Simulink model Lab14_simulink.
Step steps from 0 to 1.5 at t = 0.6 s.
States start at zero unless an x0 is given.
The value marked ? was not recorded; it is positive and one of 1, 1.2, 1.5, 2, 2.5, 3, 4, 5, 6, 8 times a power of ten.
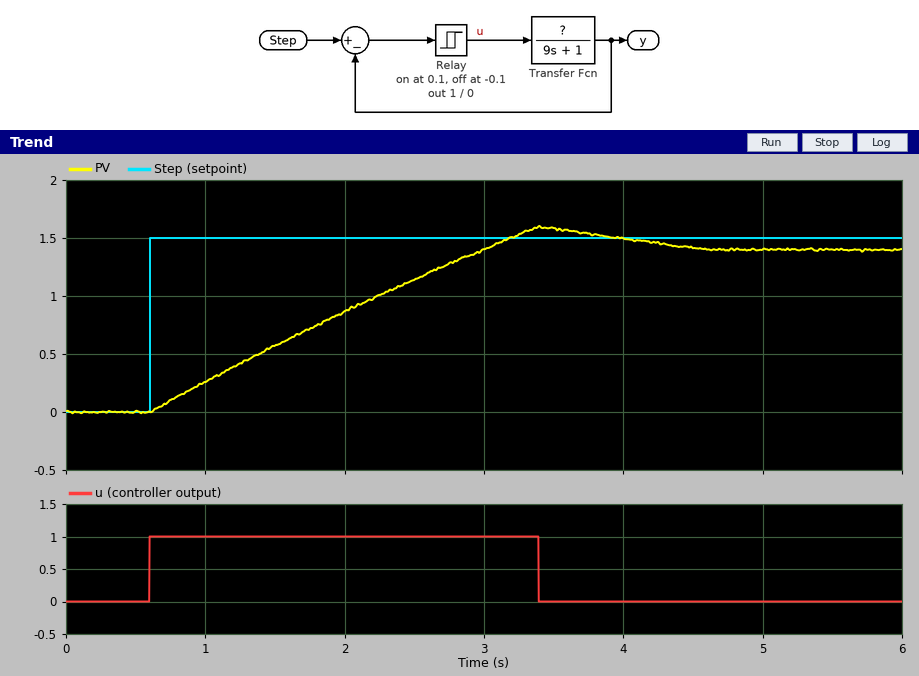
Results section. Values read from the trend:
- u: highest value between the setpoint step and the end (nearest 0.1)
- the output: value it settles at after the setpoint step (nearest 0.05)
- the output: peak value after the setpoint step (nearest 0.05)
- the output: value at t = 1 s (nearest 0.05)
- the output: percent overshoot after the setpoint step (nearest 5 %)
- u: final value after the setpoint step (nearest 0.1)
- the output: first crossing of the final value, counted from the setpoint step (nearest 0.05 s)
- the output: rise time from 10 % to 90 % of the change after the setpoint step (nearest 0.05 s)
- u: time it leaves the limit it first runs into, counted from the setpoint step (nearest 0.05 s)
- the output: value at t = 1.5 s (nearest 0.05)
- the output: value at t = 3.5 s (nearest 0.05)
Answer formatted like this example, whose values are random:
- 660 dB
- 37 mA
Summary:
- 1.0
- 1.40
- 1.60
- 0.25
- 15 %
- 0.0
- 2.40 s
- 1.90 s
- 2.80 s
- 0.55
- 1.60
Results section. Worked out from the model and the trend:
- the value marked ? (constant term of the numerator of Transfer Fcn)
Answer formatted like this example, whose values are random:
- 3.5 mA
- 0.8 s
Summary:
- 6
